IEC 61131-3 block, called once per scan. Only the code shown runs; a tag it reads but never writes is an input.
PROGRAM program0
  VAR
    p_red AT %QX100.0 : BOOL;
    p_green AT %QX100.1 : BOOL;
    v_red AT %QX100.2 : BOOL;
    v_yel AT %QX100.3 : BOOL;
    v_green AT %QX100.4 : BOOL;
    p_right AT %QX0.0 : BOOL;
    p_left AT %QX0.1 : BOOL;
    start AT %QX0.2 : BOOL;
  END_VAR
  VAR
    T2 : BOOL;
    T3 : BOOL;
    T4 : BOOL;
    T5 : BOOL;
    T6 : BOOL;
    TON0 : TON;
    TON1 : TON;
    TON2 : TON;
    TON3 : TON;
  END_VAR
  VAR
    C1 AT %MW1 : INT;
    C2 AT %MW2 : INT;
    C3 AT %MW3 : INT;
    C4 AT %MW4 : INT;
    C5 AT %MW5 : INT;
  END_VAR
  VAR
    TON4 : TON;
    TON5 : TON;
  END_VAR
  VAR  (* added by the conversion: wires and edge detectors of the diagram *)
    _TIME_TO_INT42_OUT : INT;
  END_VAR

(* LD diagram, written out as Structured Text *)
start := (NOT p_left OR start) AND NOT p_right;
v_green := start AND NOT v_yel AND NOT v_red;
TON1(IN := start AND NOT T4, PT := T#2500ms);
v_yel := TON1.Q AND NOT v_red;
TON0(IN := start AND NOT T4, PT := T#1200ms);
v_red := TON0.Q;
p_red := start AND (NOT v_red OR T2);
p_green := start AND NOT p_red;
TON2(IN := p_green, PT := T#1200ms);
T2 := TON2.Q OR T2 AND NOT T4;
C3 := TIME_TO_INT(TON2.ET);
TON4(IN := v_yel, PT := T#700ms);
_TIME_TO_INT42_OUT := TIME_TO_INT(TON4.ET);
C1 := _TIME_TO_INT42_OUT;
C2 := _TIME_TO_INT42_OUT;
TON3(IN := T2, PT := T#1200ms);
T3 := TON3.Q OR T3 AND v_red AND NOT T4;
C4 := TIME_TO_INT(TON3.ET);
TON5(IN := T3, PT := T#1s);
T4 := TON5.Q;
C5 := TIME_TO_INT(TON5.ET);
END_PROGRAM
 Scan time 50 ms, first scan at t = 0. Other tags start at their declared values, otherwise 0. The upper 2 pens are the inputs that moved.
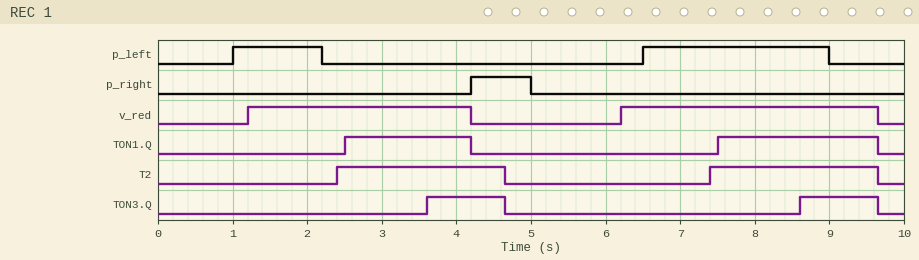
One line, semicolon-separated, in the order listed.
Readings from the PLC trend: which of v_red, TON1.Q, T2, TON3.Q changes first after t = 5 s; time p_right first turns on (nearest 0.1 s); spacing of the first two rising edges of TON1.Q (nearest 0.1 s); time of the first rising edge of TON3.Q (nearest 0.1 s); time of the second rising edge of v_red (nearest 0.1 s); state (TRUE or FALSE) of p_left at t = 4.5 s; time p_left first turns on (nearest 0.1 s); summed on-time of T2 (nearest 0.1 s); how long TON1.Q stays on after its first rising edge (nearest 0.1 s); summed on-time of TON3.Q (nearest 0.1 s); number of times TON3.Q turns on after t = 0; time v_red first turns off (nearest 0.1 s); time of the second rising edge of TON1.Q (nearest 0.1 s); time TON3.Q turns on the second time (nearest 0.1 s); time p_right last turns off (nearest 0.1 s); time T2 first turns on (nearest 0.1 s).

v_red; 4.2 s; 5.0 s; 3.6 s; 6.2 s; FALSE; 1.0 s; 4.5 s; 1.7 s; 2.1 s; 2; 4.2 s; 7.5 s; 8.6 s; 5.0 s; 2.4 s
